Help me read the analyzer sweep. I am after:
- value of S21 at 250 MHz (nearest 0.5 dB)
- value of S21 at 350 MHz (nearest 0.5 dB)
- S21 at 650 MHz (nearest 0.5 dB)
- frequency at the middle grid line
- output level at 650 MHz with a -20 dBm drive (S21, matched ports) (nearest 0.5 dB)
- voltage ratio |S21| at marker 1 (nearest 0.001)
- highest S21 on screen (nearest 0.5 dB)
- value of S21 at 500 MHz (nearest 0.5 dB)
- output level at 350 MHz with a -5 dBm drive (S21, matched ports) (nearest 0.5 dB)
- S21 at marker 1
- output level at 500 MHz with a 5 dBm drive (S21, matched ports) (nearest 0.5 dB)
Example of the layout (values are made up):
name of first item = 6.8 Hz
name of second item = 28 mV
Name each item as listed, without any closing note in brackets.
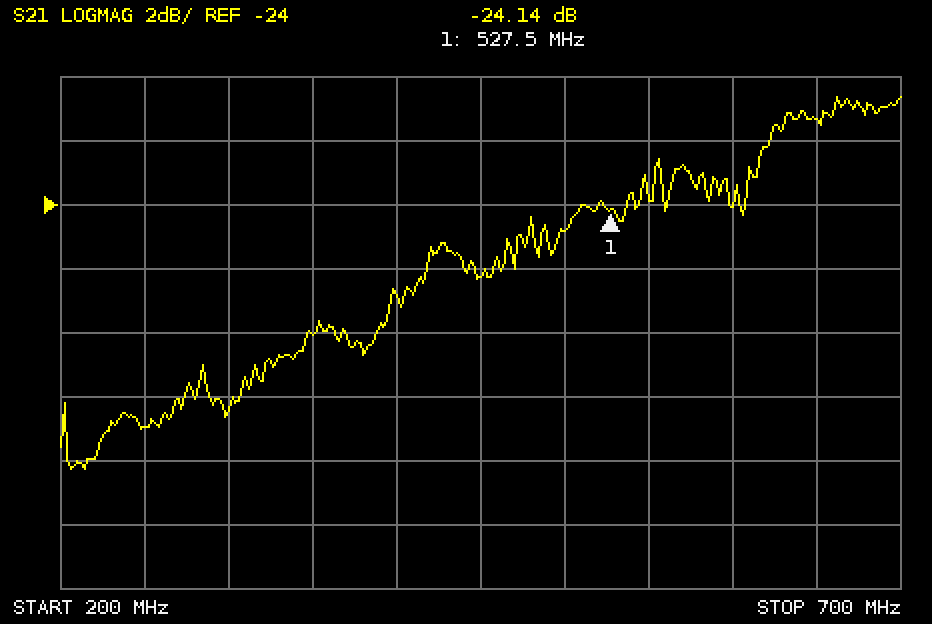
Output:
value of S21 at 250 MHz = -31.0 dB
value of S21 at 350 MHz = -28.0 dB
S21 at 650 MHz = -21.5 dB
frequency at the middle grid line = 450 MHz
output level at 650 MHz with a -20 dBm drive (S21, matched ports) = -41.5 dBm
voltage ratio |S21| at marker 1 = 0.062
highest S21 on screen = -20.5 dB
value of S21 at 500 MHz = -25.0 dB
output level at 350 MHz with a -5 dBm drive (S21, matched ports) = -33.0 dBm
S21 at marker 1 = -24.14 dB
output level at 500 MHz with a 5 dBm drive (S21, matched ports) = -20.0 dBm
